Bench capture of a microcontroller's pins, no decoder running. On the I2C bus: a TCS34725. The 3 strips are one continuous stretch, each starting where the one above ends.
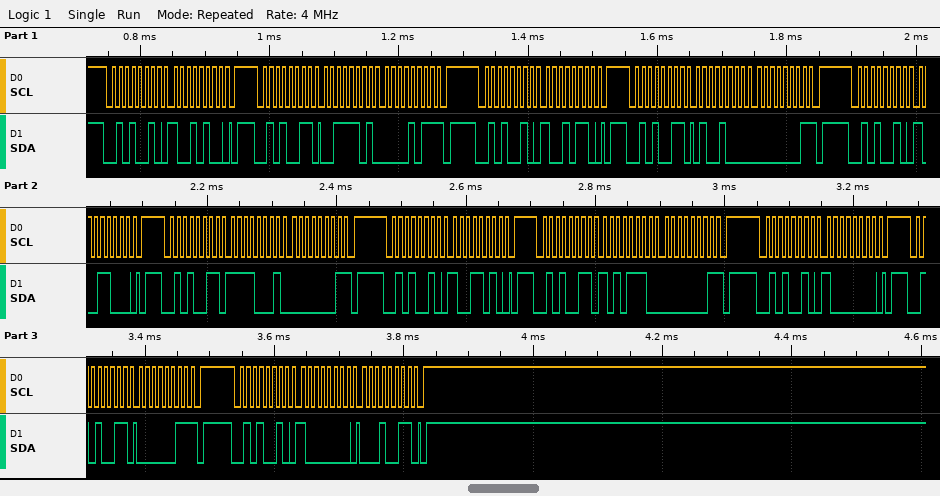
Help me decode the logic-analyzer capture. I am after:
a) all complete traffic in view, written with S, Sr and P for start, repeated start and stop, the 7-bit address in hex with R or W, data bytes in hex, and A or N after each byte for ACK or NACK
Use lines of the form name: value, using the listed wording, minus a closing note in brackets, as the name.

all complete traffic in view, written with S, Sr and P for start, repeated start and stop, the 7-bit address in hex with R or W, data bytes in hex, and A or N after each byte for ACK or NACK: S 29W A 94 A P S 29R A 3D A 0B N P S 29W A 96 A P S 29R A 48 A 01 N P S 29W A 98 A P S 29R A F1 A 01 N P S 29W A 9A A P S 29R A AE A 01 N P S 29W A 80 A P S 29R A 03 N P S 29W A 80 A 13 A P
